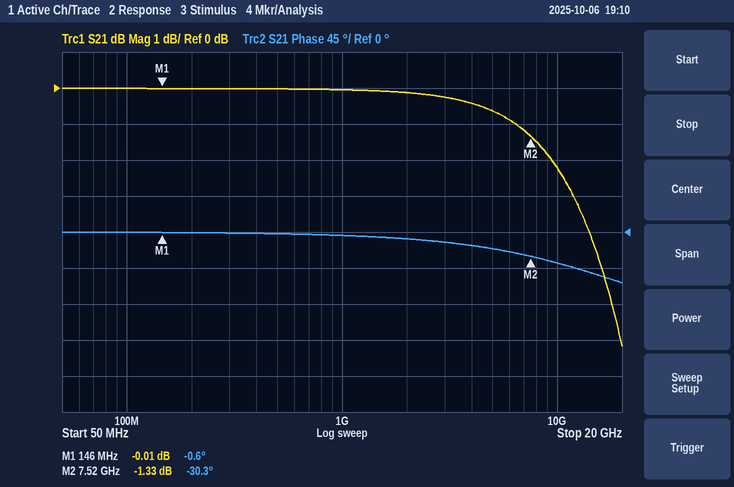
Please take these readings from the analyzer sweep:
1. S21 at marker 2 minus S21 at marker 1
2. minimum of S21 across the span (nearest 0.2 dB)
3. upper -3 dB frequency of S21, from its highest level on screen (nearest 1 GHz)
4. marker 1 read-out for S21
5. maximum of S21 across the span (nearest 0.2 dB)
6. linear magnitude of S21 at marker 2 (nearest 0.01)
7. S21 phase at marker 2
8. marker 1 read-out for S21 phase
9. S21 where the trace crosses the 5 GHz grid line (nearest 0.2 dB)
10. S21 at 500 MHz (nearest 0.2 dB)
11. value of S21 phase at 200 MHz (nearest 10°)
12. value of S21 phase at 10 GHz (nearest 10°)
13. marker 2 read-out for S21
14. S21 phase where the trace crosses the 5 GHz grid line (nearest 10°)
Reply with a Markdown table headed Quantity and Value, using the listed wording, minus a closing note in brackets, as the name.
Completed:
| Quantity | Value |
|---|---|
| S21 at marker 2 minus S21 at marker 1 | -1.32 dB |
| minimum of S21 across the span | -7.2 dB |
| upper -3 dB frequency of S21, from its highest level on screen | 12 GHz |
| marker 1 read-out for S21 | -0.01 dB |
| maximum of S21 across the span | 0.0 dB |
| linear magnitude of S21 at marker 2 | 0.86 |
| S21 phase at marker 2 | -30.3° |
| marker 1 read-out for S21 phase | -0.6° |
| S21 where the trace crosses the 5 GHz grid line | -0.6 dB |
| S21 at 500 MHz | 0.0 dB |
| value of S21 phase at 200 MHz | 0° |
| value of S21 phase at 10 GHz | -40° |
| marker 2 read-out for S21 | -1.33 dB |
| S21 phase where the trace crosses the 5 GHz grid line | -20° |
